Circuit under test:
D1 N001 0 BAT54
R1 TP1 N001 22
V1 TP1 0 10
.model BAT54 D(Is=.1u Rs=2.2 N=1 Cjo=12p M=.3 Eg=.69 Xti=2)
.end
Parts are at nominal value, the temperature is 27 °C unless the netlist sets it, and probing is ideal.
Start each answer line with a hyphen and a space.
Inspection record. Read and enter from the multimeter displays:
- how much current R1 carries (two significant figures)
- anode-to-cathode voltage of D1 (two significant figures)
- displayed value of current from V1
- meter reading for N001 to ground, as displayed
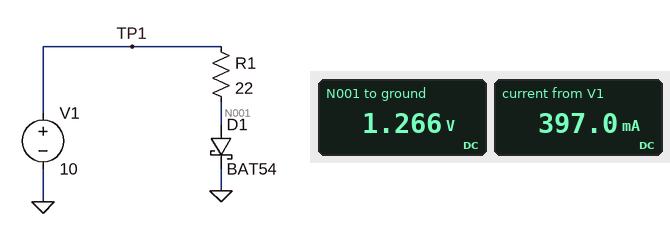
- 400 mA
- 1.3 V
- 397.0 mA
- 1.266 V
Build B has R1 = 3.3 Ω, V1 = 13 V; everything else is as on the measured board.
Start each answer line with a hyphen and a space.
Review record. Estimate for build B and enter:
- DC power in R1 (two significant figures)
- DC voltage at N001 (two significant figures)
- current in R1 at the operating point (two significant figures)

- 17 W
- 5.5 V
- 2.3 A
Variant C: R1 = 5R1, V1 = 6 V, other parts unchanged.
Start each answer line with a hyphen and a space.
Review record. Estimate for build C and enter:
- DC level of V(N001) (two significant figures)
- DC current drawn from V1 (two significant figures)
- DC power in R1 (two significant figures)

- 2.1 V
- 770 mA
- 3.0 W
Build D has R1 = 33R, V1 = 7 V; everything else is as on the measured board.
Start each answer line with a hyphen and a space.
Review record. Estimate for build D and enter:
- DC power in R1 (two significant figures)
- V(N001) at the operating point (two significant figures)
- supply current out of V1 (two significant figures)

- 1.2 W
- 790 mV
- 190 mA
